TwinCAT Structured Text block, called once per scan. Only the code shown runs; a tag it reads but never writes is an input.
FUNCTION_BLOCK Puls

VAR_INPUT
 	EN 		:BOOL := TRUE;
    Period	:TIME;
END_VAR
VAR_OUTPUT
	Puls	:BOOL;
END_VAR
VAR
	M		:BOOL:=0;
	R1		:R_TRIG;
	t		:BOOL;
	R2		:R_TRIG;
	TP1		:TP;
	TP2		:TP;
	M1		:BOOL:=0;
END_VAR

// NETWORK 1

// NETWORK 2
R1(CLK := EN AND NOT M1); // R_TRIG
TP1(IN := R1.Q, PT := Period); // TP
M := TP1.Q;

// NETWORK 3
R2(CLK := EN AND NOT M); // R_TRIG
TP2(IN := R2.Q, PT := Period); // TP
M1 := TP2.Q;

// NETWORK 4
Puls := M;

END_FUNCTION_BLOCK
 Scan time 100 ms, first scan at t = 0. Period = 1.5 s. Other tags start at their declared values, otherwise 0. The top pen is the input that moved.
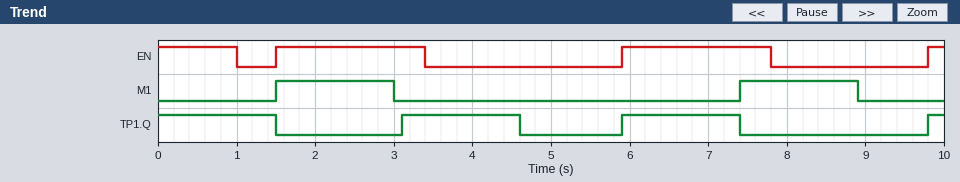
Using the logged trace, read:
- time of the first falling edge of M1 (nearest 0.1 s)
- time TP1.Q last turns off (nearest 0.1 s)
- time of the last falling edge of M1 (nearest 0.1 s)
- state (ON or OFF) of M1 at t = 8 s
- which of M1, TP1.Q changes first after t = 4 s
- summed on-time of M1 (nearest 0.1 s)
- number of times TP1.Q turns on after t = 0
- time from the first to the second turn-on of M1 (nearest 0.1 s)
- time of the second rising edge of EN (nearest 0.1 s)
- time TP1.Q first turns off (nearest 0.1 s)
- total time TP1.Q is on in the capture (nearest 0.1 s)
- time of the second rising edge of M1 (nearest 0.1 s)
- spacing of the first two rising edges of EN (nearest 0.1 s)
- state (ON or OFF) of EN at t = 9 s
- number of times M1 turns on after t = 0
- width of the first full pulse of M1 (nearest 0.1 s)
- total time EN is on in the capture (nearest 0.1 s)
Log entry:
3.0 s
7.4 s
8.9 s
ON
TP1.Q
3.0 s
3
5.9 s
5.9 s
1.5 s
4.7 s
7.4 s
4.4 s
OFF
2
1.5 s
5.0 s
